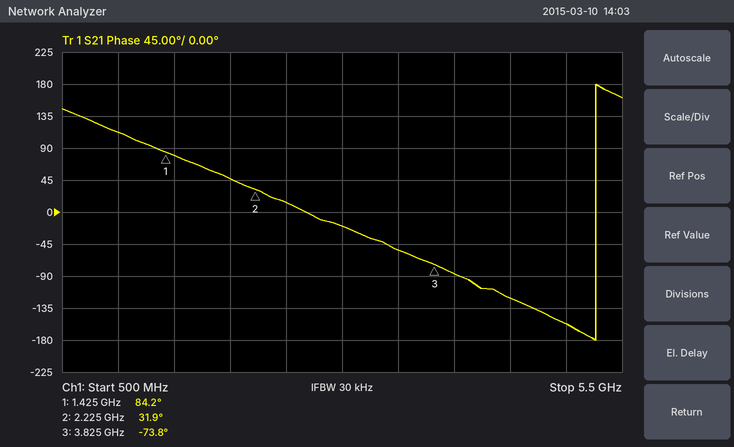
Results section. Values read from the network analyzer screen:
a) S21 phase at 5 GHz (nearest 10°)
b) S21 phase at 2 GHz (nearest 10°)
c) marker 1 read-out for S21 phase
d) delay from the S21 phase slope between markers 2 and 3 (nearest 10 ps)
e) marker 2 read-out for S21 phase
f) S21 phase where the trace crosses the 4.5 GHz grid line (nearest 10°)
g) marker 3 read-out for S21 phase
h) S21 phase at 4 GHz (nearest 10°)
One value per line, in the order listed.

-160°
50°
84.2°
180 ps
31.9°
-120°
-73.8°
-90°
